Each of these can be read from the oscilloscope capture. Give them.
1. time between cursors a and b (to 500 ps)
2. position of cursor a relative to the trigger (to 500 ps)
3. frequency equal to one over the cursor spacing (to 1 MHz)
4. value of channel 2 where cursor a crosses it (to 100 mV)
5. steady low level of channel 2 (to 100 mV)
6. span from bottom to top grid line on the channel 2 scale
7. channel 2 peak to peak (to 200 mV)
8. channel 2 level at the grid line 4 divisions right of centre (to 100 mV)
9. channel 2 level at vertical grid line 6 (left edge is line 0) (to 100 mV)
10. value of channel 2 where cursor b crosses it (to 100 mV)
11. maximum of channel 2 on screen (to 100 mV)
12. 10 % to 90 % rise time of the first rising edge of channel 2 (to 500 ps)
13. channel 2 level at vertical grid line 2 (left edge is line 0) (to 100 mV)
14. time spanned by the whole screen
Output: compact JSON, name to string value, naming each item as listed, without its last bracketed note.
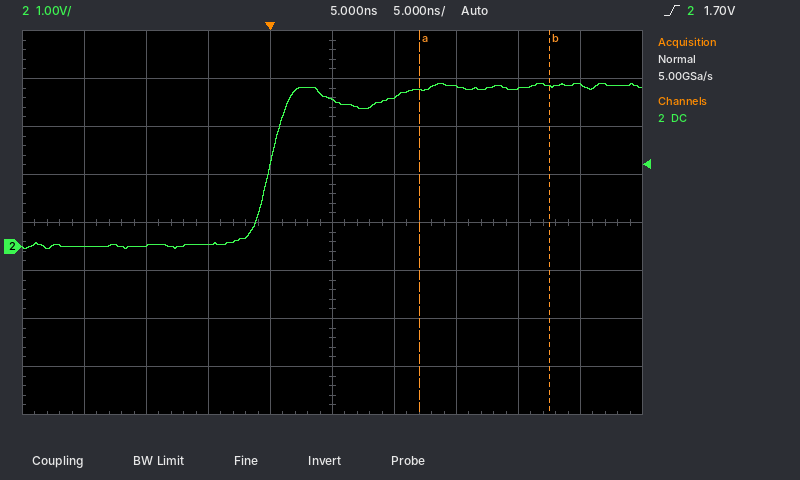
{"time between cursors a and b": "10.5 ns", "position of cursor a relative to the trigger": "+12.0 ns", "frequency equal to one over the cursor spacing": "95 MHz", "value of channel 2 where cursor a crosses it": "3.3 V", "steady low level of channel 2": "0.0 V", "span from bottom to top grid line on the channel 2 scale": "8 V", "channel 2 peak to peak": "3.4 V", "channel 2 level at the grid line 4 divisions right of centre": "3.4 V", "channel 2 level at vertical grid line 6 (left edge is line 0)": "3.1 V", "value of channel 2 where cursor b crosses it": "3.3 V", "maximum of channel 2 on screen": "3.4 V", "10 % to 90 % rise time of the first rising edge of channel 2": "3.0 ns", "channel 2 level at vertical grid line 2 (left edge is line 0)": "0.0 V", "time spanned by the whole screen": "50 ns"}
